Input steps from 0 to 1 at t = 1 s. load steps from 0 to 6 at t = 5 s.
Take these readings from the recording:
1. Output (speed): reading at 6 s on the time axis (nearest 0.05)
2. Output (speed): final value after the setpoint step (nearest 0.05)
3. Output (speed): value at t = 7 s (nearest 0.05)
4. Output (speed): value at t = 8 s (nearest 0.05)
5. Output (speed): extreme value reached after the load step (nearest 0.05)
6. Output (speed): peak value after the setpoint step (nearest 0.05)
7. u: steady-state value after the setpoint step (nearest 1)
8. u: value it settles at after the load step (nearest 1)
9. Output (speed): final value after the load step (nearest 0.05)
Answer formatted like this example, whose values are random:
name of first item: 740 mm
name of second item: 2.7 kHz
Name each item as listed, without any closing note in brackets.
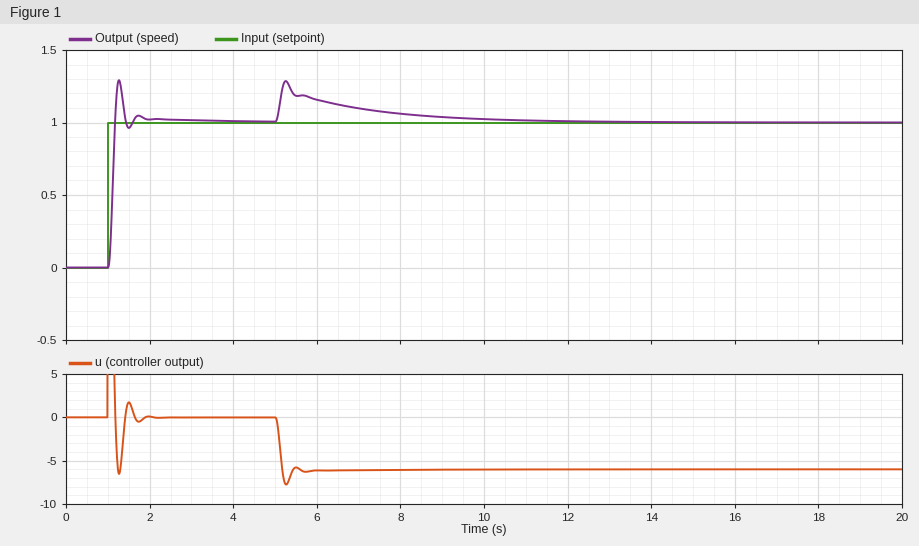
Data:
Output (speed): reading at 6 s on the time axis: 1.15
Output (speed): final value after the setpoint step: 1.00
Output (speed): value at t = 7 s: 1.10
Output (speed): value at t = 8 s: 1.05
Output (speed): extreme value reached after the load step: 1.30
Output (speed): peak value after the setpoint step: 1.30
u: steady-state value after the setpoint step: 0
u: value it settles at after the load step: -6
Output (speed): final value after the load step: 1.00
